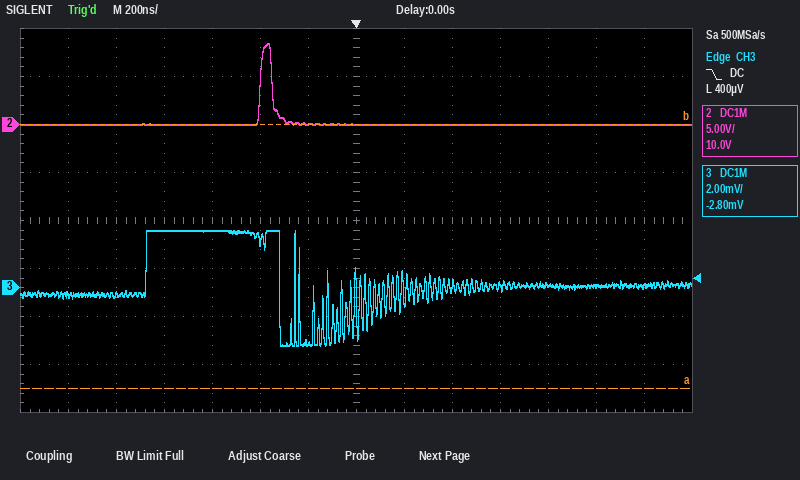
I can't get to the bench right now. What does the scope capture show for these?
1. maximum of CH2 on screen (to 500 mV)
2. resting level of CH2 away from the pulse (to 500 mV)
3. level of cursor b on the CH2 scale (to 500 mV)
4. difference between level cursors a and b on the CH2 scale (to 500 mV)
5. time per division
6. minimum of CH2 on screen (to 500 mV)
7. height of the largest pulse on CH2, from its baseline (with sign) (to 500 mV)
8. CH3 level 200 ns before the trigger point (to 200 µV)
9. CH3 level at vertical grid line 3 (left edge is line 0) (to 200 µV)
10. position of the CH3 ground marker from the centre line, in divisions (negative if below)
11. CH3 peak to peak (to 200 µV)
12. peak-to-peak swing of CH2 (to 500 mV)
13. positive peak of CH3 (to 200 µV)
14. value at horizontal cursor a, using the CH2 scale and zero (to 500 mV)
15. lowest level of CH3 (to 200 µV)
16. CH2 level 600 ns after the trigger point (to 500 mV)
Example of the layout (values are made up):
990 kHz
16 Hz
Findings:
8.5 V
0.0 V
0.0 V
27.5 V
200 ns
0.0 V
+8.5 V
-2.2 mV
2.4 mV
-1.4 div
4.8 mV
8.5 V
2.4 mV
-27.5 V
-2.4 mV
0.0 V
